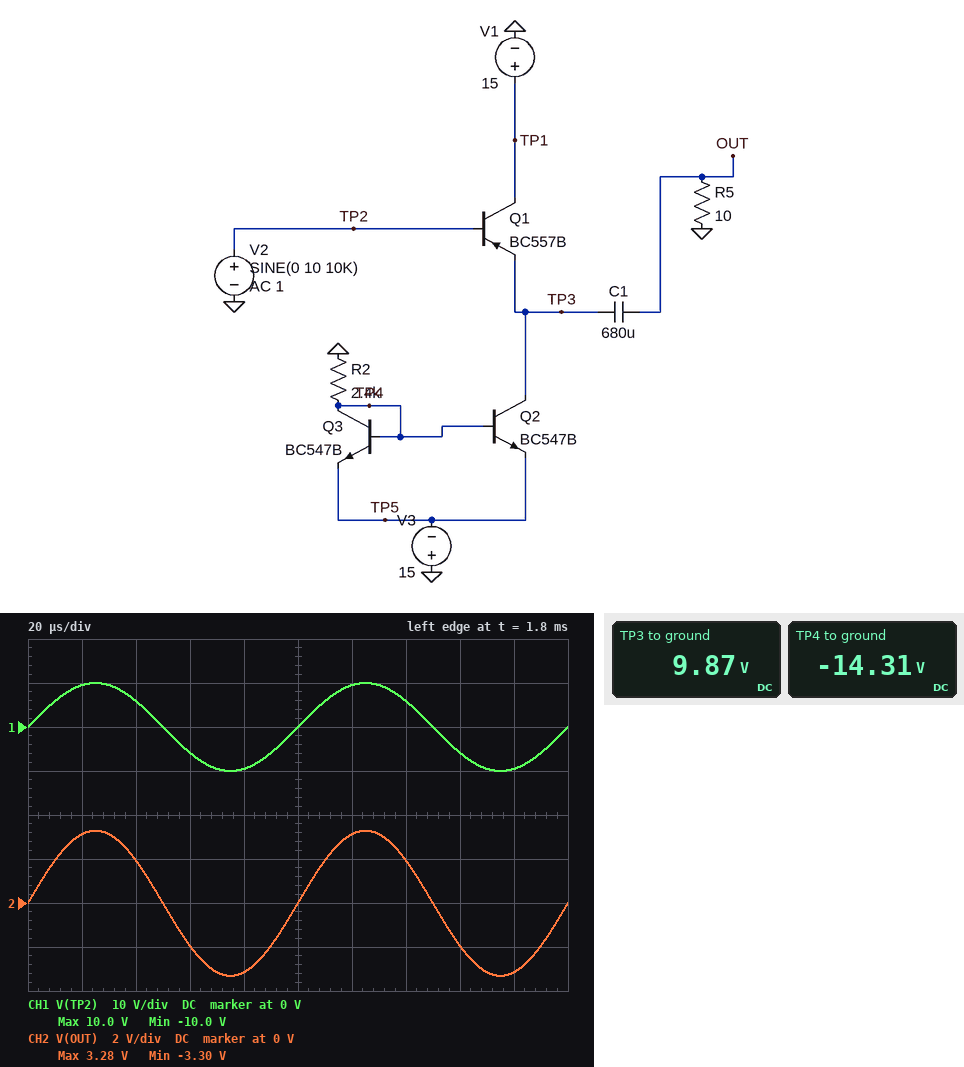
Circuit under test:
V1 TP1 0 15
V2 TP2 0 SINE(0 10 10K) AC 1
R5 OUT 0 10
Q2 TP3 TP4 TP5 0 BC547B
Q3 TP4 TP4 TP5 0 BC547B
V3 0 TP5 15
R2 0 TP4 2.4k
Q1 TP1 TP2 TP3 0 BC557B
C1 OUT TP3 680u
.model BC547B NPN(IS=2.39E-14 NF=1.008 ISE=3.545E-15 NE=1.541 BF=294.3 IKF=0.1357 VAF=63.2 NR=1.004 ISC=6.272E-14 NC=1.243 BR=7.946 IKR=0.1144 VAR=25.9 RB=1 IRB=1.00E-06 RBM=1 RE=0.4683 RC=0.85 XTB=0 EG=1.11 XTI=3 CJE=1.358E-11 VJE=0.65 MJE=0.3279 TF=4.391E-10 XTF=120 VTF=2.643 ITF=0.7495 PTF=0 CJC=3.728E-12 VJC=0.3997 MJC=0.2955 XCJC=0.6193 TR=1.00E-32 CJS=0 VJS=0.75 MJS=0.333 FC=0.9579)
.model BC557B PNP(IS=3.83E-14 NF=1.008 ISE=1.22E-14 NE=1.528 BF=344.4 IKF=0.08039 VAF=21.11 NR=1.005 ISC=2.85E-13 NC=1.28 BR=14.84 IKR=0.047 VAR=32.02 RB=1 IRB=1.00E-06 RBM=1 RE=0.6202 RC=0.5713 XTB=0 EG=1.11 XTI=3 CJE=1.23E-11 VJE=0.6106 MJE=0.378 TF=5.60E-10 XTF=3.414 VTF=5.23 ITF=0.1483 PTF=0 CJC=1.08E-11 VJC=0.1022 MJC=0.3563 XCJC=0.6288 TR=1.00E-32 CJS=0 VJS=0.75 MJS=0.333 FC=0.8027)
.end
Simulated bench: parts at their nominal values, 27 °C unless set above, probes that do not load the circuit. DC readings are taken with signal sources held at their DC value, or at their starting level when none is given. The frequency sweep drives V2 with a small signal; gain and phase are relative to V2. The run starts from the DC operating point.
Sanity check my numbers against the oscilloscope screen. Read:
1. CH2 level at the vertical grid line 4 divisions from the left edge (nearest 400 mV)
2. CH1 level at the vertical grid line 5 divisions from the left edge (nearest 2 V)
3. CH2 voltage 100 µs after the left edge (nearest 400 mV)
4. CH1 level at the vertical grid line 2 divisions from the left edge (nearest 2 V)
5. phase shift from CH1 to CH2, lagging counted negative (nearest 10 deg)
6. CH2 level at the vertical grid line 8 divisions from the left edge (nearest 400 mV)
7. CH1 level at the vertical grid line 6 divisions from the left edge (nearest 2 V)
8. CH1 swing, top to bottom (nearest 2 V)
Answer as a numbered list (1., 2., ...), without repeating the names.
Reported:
1. -3.2 V
2. 0 V
3. 0 V
4. 6 V
5. 0 deg
6. -2.0 V
7. 10 V
8. 20 V
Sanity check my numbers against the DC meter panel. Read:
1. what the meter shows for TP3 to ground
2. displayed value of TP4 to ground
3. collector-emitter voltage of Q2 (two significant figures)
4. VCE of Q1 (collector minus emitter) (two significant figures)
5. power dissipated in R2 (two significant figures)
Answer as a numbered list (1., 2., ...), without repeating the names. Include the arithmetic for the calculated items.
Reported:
1. 9.87 V
2. -14.31 V
3. 9.87 V - (-15 V) = 25 V
4. 15 V - 9.87 V = 5.1 V
5. (0 V - (-14.31 V))^2 / 2.4 kΩ = 85 mW
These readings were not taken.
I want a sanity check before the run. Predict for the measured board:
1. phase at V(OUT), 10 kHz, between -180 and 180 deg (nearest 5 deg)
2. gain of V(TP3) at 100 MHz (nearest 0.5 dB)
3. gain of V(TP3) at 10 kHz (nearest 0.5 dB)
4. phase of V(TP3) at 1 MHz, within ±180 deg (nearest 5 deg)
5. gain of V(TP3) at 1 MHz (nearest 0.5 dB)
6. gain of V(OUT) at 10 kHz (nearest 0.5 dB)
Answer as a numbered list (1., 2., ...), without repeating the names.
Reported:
1. 0 deg
2. -8.0 dB
3. -9.5 dB
4. 0 deg
5. -9.5 dB
6. -9.5 dB
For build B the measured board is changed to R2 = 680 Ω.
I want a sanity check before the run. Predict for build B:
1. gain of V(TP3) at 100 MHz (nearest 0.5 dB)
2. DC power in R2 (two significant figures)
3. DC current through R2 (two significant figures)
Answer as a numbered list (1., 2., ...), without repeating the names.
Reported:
1. -8.0 dB
2. 300 mW
3. 21 mA
